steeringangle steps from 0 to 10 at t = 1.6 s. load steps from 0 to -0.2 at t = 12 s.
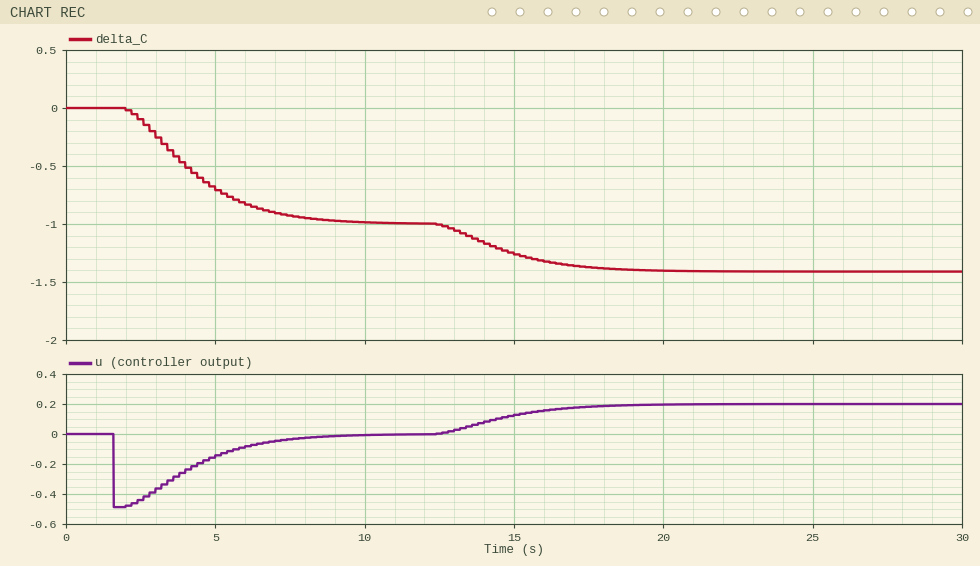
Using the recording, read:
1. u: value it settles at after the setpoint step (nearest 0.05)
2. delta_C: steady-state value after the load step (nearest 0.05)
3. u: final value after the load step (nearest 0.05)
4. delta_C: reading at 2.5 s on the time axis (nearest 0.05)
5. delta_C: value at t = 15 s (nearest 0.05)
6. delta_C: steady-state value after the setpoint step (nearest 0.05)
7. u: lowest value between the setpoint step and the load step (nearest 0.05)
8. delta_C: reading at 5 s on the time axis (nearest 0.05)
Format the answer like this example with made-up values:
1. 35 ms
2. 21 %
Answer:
1. 0.00
2. -1.40
3. 0.20
4. -0.10
5. -1.25
6. -1.00
7. -0.50
8. -0.70
